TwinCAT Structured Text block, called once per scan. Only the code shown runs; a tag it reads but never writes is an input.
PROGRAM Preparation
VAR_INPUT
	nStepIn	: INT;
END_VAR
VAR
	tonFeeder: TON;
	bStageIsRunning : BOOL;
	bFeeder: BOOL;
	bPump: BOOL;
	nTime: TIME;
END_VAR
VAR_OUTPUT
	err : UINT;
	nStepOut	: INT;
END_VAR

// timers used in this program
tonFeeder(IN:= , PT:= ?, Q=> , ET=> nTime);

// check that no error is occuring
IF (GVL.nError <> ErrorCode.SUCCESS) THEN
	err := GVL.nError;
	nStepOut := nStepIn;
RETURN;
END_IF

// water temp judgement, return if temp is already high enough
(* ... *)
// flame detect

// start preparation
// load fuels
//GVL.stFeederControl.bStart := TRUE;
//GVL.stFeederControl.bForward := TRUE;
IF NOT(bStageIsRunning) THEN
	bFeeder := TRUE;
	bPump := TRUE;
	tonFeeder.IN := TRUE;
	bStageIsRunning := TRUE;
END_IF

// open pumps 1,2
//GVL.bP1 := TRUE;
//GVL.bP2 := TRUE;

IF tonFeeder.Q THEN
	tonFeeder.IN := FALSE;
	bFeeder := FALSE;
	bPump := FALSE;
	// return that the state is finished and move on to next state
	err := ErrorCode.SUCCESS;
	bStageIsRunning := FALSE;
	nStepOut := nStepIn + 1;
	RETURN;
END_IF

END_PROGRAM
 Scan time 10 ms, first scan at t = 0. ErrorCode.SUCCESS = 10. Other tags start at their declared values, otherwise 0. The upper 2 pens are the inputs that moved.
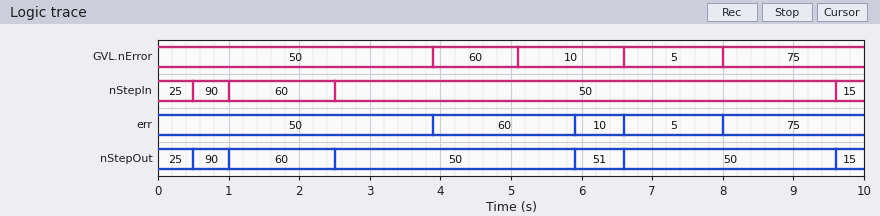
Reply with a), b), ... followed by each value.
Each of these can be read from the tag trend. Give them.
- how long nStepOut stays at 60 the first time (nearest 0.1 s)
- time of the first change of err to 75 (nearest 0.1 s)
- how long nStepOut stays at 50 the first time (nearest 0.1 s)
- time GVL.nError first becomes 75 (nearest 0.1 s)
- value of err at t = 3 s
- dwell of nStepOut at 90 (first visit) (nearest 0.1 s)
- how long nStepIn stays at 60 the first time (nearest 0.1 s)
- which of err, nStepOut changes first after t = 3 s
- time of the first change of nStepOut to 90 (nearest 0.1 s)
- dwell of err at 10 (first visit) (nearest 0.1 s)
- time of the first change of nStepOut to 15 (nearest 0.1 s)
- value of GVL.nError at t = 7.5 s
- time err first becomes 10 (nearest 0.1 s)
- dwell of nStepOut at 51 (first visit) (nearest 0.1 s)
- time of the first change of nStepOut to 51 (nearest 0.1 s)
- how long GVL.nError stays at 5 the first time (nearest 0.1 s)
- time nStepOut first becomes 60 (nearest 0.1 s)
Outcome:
a) 1.5 s
b) 8.0 s
c) 3.4 s
d) 8.0 s
e) 50
f) 0.5 s
g) 1.5 s
h) err
i) 0.5 s
j) 0.7 s
k) 9.6 s
l) 5
m) 5.9 s
n) 0.7 s
o) 5.9 s
p) 1.4 s
q) 1.0 s
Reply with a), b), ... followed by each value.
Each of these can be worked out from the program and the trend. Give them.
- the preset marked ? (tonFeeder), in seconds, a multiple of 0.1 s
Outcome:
a) 0.8 s
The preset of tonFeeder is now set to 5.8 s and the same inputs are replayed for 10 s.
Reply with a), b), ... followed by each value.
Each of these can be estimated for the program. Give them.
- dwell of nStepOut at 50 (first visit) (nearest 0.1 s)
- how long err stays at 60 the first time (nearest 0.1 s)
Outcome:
a) 7.1 s
b) 2.7 s
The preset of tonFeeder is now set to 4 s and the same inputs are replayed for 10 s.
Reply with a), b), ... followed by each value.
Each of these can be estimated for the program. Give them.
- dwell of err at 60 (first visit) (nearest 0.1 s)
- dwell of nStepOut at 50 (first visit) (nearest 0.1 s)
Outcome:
a) 2.7 s
b) 7.1 s
